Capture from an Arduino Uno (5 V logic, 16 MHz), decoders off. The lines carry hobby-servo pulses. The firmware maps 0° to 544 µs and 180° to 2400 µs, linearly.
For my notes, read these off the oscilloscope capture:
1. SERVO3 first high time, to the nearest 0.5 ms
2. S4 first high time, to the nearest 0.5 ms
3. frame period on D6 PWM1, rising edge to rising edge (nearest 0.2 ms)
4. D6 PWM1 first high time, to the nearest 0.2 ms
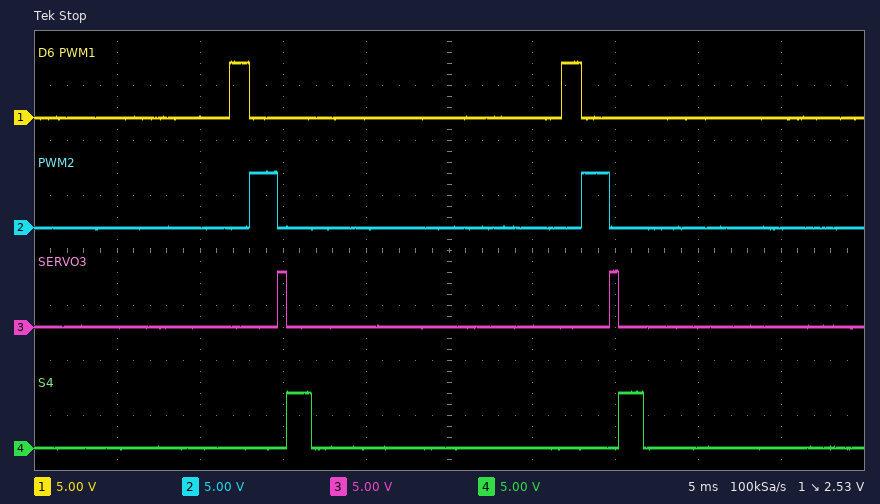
0.5 ms
1.5 ms
20.0 ms
1.2 ms
